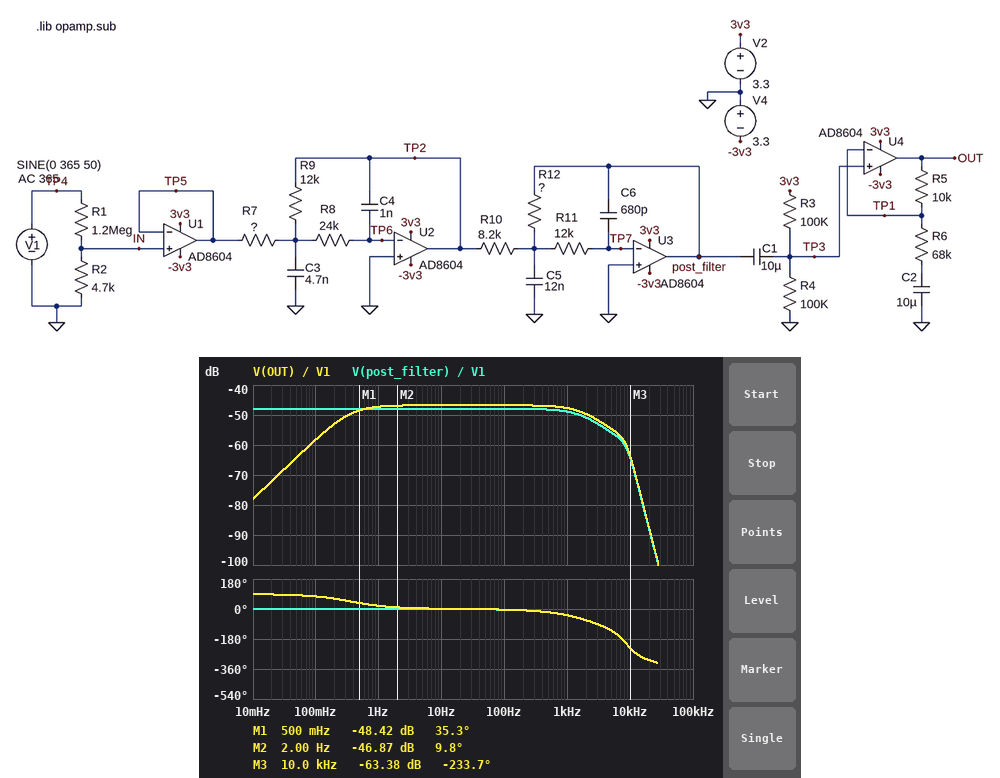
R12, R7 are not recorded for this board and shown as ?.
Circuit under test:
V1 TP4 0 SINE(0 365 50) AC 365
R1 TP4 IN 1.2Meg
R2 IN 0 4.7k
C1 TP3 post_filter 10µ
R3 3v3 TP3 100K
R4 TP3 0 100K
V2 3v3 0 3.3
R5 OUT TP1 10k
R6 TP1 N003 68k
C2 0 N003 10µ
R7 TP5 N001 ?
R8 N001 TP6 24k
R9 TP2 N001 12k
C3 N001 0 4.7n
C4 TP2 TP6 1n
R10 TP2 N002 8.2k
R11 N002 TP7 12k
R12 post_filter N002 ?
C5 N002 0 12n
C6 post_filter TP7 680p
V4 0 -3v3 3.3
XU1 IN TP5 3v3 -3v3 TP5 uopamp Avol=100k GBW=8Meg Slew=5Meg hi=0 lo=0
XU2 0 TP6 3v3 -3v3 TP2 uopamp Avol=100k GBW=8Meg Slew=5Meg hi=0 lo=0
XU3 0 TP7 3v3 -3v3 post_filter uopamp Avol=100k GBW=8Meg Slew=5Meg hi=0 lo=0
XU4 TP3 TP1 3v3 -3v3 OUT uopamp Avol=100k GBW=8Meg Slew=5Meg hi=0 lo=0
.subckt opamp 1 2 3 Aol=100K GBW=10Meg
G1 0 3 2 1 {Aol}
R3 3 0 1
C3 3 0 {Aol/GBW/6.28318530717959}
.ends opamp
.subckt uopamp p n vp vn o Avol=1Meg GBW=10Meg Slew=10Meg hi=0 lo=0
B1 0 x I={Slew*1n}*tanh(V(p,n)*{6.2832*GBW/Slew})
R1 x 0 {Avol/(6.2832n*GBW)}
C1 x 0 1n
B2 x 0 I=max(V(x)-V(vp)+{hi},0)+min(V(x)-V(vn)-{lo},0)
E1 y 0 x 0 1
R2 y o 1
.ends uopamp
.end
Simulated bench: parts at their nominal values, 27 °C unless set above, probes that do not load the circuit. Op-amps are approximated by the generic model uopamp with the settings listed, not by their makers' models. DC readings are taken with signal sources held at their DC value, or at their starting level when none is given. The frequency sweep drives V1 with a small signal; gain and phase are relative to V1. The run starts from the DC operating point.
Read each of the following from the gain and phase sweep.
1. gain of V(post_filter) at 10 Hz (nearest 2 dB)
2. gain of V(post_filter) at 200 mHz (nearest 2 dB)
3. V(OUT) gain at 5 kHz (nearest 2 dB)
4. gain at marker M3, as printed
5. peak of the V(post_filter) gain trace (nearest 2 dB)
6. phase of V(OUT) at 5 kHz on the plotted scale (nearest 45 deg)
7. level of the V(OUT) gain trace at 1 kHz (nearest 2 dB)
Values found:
-48 dB
-48 dB
-54 dB
-63.38 dB
-48 dB
-135 deg
-48 dB
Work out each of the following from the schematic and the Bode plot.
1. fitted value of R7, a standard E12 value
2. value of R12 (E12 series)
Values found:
4.7 kΩ
3.3 kΩ
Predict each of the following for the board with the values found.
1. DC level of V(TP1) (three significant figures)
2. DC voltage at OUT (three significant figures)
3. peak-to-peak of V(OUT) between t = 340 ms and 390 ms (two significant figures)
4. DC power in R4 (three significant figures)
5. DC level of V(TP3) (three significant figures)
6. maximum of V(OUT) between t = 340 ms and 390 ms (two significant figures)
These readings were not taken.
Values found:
1.65 V
1.65 V
3.1 V
27.2 µW
1.65 V
3.2 V
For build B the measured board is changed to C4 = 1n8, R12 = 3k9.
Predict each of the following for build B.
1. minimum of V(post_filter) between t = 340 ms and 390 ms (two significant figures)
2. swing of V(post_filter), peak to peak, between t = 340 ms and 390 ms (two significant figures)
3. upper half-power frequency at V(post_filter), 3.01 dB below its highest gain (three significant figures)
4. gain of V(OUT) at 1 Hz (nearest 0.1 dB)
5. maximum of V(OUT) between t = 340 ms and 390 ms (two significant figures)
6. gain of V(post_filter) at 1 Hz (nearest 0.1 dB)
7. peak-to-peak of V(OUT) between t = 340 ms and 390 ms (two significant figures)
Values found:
-1.6 V
3.1 V
1.01 kHz
-45.8 dB
3.3 V
-46.5 dB
3.5 V
